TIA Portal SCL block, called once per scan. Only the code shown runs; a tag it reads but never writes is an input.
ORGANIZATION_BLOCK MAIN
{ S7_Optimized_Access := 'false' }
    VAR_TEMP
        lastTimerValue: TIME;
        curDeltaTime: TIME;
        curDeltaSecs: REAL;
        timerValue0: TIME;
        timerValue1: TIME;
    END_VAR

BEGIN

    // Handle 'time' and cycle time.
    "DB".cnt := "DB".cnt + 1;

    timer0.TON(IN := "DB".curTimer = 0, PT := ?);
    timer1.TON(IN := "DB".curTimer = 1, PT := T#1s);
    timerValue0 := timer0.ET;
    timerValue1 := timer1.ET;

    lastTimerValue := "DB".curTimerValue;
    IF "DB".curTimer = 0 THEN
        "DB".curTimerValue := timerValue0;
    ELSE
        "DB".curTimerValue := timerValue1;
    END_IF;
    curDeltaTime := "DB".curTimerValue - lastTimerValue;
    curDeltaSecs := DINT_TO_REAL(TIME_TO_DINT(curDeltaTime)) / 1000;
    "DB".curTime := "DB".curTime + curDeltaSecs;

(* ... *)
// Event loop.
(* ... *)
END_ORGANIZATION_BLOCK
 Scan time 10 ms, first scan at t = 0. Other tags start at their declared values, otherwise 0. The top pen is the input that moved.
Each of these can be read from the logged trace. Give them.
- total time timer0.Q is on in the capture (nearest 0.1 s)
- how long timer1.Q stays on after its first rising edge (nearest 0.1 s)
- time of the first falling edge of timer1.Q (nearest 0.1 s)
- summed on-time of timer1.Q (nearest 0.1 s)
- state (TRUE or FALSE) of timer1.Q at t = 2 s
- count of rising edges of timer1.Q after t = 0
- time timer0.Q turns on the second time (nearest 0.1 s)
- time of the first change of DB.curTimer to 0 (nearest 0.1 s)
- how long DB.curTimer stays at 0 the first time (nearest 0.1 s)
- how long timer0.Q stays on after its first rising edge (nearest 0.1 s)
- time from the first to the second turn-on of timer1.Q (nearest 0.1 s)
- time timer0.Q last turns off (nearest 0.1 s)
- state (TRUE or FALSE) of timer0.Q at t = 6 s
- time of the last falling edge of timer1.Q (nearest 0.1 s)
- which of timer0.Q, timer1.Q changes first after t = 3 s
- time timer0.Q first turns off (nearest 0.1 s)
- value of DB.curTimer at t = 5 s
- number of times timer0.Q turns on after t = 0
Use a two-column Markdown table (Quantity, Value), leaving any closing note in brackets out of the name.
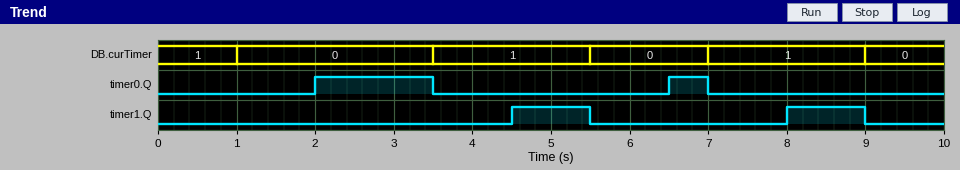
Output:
| Quantity | Value |
|---|---|
| total time timer0.Q is on in the capture | 2.0 s |
| how long timer1.Q stays on after its first rising edge | 1.0 s |
| time of the first falling edge of timer1.Q | 5.5 s |
| summed on-time of timer1.Q | 2.0 s |
| state (TRUE or FALSE) of timer1.Q at t = 2 s | FALSE |
| count of rising edges of timer1.Q after t = 0 | 2 |
| time timer0.Q turns on the second time | 6.5 s |
| time of the first change of DB.curTimer to 0 | 1.0 s |
| how long DB.curTimer stays at 0 the first time | 2.5 s |
| how long timer0.Q stays on after its first rising edge | 1.5 s |
| time from the first to the second turn-on of timer1.Q | 3.5 s |
| time timer0.Q last turns off | 7.0 s |
| state (TRUE or FALSE) of timer0.Q at t = 6 s | FALSE |
| time of the last falling edge of timer1.Q | 9.0 s |
| which of timer0.Q, timer1.Q changes first after t = 3 s | timer0.Q |
| time timer0.Q first turns off | 3.5 s |
| value of DB.curTimer at t = 5 s | 1 |
| number of times timer0.Q turns on after t = 0 | 2 |
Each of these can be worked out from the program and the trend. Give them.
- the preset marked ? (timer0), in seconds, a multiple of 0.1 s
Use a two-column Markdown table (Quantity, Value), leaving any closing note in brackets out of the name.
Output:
| Quantity | Value |
|---|---|
| the preset marked ? (timer0), in seconds, a multiple of 0.1 s | 1.0 s |
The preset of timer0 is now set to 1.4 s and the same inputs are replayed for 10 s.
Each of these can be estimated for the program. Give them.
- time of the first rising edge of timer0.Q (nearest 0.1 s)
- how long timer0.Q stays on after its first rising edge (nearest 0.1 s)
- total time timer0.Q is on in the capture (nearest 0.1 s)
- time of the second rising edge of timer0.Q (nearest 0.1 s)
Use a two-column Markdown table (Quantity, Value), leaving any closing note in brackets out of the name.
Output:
| Quantity | Value |
|---|---|
| time of the first rising edge of timer0.Q | 2.4 s |
| how long timer0.Q stays on after its first rising edge | 1.1 s |
| total time timer0.Q is on in the capture | 1.2 s |
| time of the second rising edge of timer0.Q | 6.9 s |
